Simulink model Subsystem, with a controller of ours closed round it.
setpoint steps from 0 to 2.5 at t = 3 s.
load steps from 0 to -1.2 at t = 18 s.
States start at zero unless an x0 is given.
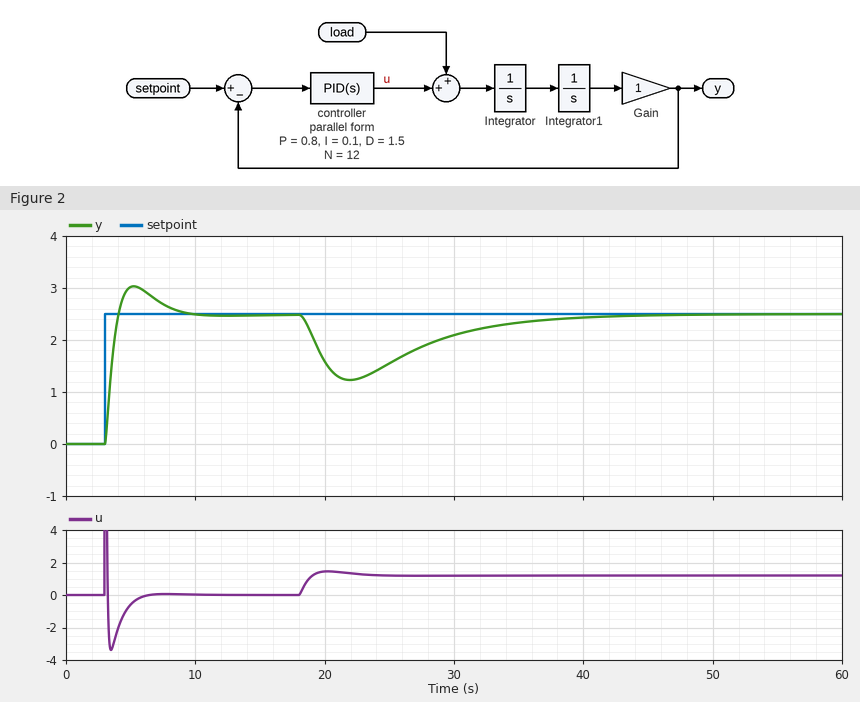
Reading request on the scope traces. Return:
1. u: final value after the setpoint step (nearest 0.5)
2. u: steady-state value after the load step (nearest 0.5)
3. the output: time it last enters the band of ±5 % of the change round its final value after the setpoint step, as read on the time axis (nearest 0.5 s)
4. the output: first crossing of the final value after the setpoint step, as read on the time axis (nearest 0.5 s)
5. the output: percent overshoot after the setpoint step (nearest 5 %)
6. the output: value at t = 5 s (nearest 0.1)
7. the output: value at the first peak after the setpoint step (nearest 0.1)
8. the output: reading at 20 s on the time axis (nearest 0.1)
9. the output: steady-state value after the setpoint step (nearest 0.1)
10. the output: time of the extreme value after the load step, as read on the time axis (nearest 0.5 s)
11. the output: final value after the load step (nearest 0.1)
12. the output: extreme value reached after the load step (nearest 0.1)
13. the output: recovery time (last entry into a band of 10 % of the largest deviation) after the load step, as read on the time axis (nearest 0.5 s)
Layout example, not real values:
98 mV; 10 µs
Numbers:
0.0; 1.0; 8.0 s; 4.0 s; 20 %; 3.0; 3.0; 1.6; 2.5; 22.0 s; 2.5; 1.2; 36.5 s
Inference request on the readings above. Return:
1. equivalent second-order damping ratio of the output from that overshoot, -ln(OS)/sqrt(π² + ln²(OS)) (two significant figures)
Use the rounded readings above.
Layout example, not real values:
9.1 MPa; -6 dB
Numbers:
0.46
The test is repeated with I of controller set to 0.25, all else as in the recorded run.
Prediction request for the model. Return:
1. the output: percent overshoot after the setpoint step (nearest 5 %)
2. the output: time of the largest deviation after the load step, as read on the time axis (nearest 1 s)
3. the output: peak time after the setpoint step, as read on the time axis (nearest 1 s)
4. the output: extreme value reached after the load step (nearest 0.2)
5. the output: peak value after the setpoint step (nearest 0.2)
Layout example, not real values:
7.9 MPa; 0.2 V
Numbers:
25 %; 21 s; 5 s; 1.4; 3.2
